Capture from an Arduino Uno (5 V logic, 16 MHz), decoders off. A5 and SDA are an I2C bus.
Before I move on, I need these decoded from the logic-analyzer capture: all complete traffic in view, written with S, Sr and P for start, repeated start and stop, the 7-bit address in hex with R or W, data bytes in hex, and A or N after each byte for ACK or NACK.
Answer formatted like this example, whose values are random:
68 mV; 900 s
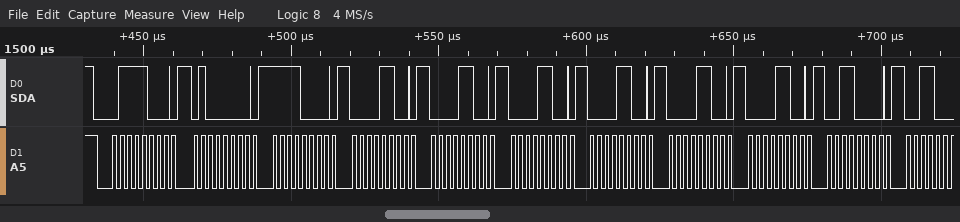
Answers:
S 3CW A 40 A F0 A 0C A 0C A 0C A 0C A 0C A 0C A 30 A
